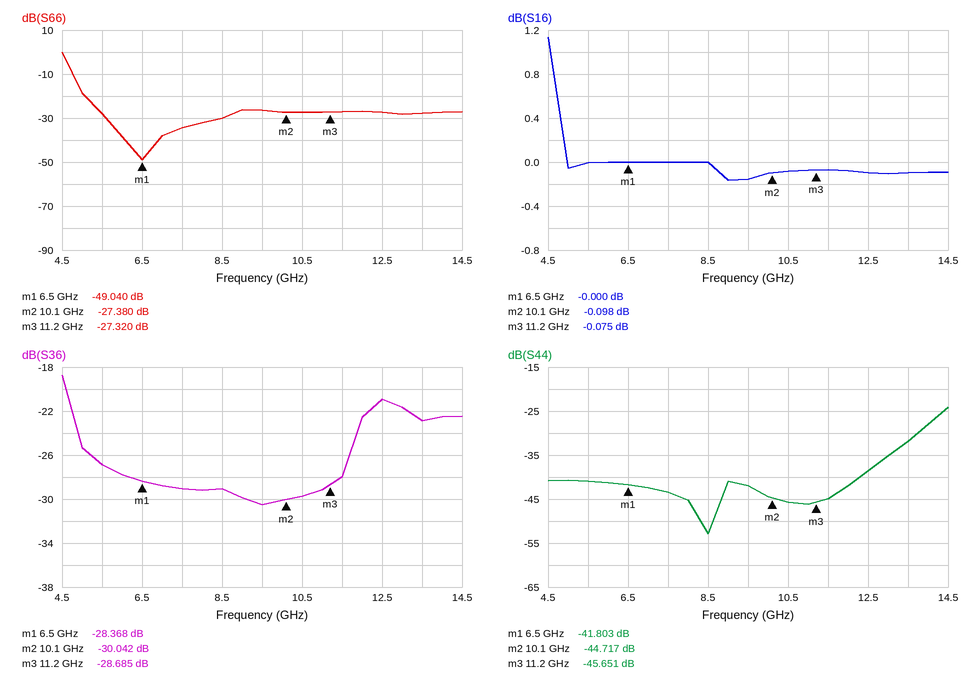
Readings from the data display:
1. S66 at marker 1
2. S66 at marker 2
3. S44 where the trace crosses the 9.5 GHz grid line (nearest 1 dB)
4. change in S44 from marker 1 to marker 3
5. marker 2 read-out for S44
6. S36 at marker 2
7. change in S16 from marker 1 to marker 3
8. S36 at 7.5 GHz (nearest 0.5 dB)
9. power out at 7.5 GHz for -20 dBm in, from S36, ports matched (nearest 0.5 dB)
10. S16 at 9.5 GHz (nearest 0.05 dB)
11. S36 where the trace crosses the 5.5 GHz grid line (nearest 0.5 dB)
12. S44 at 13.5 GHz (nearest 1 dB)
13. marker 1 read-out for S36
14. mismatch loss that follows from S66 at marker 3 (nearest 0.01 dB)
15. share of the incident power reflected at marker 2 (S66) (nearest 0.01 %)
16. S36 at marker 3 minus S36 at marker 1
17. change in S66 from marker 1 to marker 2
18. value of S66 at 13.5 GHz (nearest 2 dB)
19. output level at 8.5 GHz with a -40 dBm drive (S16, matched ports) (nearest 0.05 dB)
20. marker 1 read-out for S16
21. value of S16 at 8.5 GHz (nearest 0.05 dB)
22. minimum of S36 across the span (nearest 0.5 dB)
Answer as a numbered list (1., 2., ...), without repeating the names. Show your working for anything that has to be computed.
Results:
1. -49.040 dB
2. -27.380 dB
3. -42 dB
4. -45.651 − (-41.803) = -3.848 dB
5. -44.717 dB
6. -30.042 dB
7. -0.075 − (-0) = -0.075 dB
8. -29.0 dB
9. -20 dBm + (-29.0 dB) = -49.0 dBm
10. -0.15 dB
11. -27.0 dB
12. -32 dB
13. -28.368 dB
14. −10 log10(1 − 10^(-27.32/10)) ≈ 0.01 dB
15. 10^(-27.38/10) ≈ 0.18 %
16. -28.685 − (-28.368) = -0.317 dB
17. -27.38 − (-49.04) = 21.660 dB
18. -28 dB
19. -40 dBm + (0.00 dB) = -40.00 dBm
20. -0.000 dB
21. 0.00 dB
22. -30.5 dB
